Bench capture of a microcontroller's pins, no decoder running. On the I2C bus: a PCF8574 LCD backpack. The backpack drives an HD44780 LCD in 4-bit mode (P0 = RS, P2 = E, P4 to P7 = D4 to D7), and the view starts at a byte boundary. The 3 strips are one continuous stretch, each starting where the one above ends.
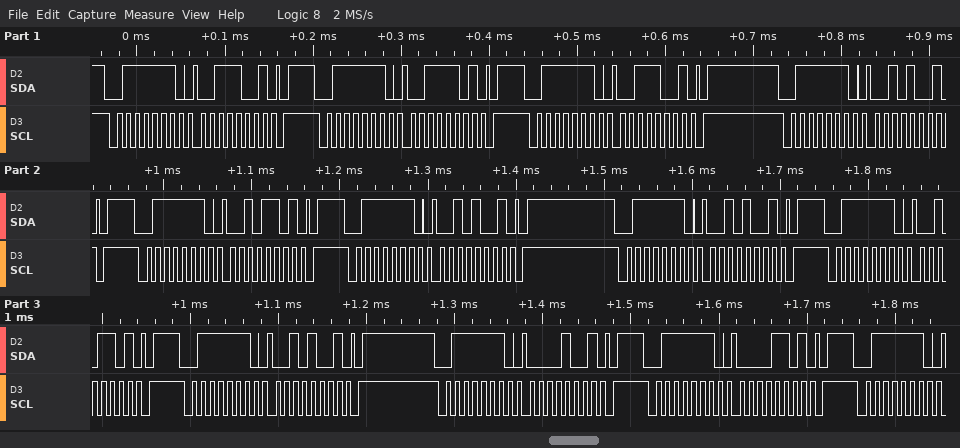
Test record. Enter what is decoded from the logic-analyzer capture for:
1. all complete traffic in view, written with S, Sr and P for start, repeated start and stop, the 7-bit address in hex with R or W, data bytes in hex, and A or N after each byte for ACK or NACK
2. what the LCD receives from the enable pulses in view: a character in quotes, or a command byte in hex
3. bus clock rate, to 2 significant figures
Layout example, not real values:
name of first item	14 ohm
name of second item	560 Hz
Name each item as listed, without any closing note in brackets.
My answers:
all complete traffic in view, written with S, Sr and P for start, repeated start and stop, the 7-bit address in hex with R or W, data bytes in hex, and A or N after each byte for ACK or NACK	S 3FW A 39 A P S 3FW A 3D A P S 3FW A 39 A P S 3FW A 29 A P S 3FW A 2D A P S 3FW A 29 A P S 3FW A 29 A P S 3FW A 2D A P S 3FW A 29 A P S 3FW A 09 A P S 3FW A 0D A P S 3FW A
what the LCD receives from the enable pulses in view: a character in quotes, or a command byte in hex	'2'
bus clock rate, to 2 significant figures	100 kHz
